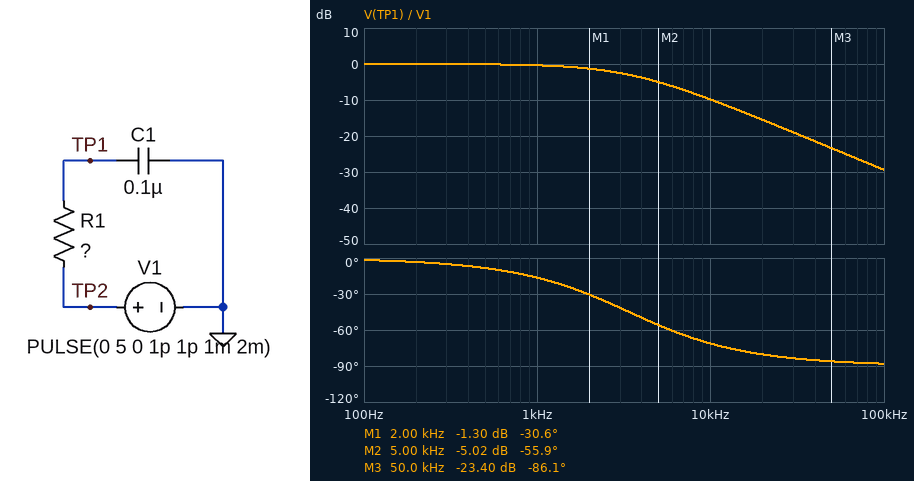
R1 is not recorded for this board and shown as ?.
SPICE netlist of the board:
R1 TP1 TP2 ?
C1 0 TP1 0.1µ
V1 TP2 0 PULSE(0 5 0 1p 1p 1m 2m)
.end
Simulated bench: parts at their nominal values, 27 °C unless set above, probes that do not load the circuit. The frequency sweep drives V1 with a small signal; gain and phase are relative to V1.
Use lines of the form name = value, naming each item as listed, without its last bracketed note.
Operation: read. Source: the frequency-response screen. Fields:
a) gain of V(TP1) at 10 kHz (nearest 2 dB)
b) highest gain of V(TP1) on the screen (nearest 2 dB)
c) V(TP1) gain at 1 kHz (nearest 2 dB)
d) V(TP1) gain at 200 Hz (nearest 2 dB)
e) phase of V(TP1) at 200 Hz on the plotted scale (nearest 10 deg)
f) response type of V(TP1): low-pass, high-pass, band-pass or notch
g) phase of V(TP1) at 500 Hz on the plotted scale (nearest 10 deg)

gain of V(TP1) at 10 kHz = -10 dB
highest gain of V(TP1) on the screen = 0 dB
V(TP1) gain at 1 kHz = 0 dB
V(TP1) gain at 200 Hz = 0 dB
phase of V(TP1) at 200 Hz on the plotted scale = 0 deg
response type of V(TP1): low-pass, high-pass, band-pass or notch = low-pass
phase of V(TP1) at 500 Hz on the plotted scale = -10 deg
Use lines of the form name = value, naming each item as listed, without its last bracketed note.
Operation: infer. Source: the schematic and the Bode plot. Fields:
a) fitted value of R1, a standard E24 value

fitted value of R1, a standard E24 value = 470 Ω
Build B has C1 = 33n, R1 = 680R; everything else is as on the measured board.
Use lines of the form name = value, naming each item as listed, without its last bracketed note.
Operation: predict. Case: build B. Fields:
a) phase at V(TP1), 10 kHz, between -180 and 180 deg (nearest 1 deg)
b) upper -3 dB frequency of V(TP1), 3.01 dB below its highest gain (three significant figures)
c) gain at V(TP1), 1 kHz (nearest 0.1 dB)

phase at V(TP1), 10 kHz, between -180 and 180 deg = -55 deg
upper -3 dB frequency of V(TP1), 3.01 dB below its highest gain = 7.09 kHz
gain at V(TP1), 1 kHz = -0.1 dB
